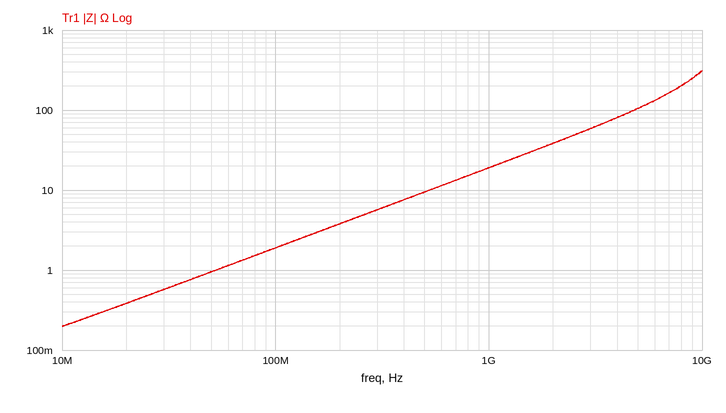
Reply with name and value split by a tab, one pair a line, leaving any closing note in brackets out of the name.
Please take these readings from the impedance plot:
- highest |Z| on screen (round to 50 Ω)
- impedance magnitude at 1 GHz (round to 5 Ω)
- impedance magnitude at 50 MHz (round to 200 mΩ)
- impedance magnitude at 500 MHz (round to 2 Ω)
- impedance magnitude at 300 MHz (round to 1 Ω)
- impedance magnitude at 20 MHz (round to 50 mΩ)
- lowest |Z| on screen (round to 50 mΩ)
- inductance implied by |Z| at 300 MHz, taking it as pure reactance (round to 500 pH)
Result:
highest |Z| on screen	300 Ω
impedance magnitude at 1 GHz	20 Ω
impedance magnitude at 50 MHz	1.0 Ω
impedance magnitude at 500 MHz	10 Ω
impedance magnitude at 300 MHz	6 Ω
impedance magnitude at 20 MHz	400 mΩ
lowest |Z| on screen	200 mΩ
inductance implied by |Z| at 300 MHz, taking it as pure reactance	3.0 nH
